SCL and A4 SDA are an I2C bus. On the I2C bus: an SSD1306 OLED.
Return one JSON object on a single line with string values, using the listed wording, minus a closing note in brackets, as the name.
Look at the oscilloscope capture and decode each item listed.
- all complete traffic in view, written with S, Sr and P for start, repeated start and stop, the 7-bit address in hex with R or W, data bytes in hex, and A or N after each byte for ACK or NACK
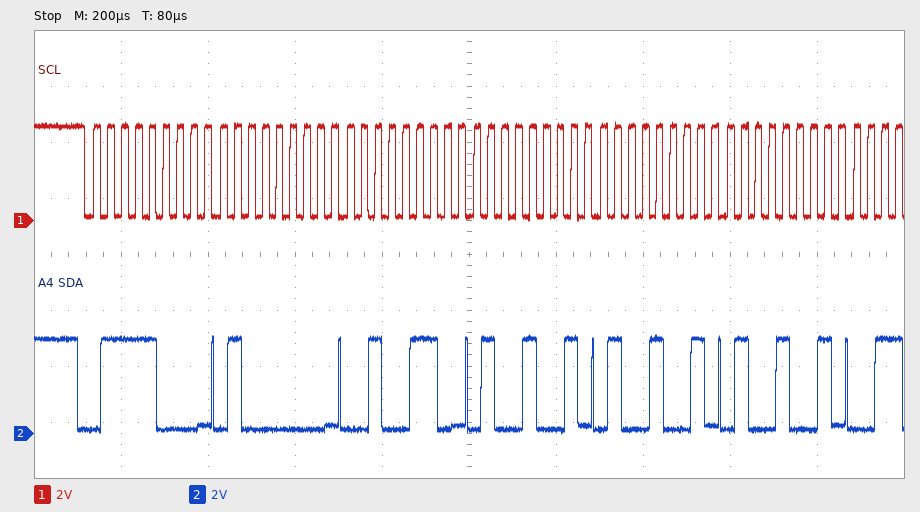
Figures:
{"all complete traffic in view, written with S, Sr and P for start, repeated start and stop, the 7-bit address in hex with R or W, data bytes in hex, and A or N after each byte for ACK or NACK": "S 3CW A 40 A 26 A 49 A 49 A 49 A"}
